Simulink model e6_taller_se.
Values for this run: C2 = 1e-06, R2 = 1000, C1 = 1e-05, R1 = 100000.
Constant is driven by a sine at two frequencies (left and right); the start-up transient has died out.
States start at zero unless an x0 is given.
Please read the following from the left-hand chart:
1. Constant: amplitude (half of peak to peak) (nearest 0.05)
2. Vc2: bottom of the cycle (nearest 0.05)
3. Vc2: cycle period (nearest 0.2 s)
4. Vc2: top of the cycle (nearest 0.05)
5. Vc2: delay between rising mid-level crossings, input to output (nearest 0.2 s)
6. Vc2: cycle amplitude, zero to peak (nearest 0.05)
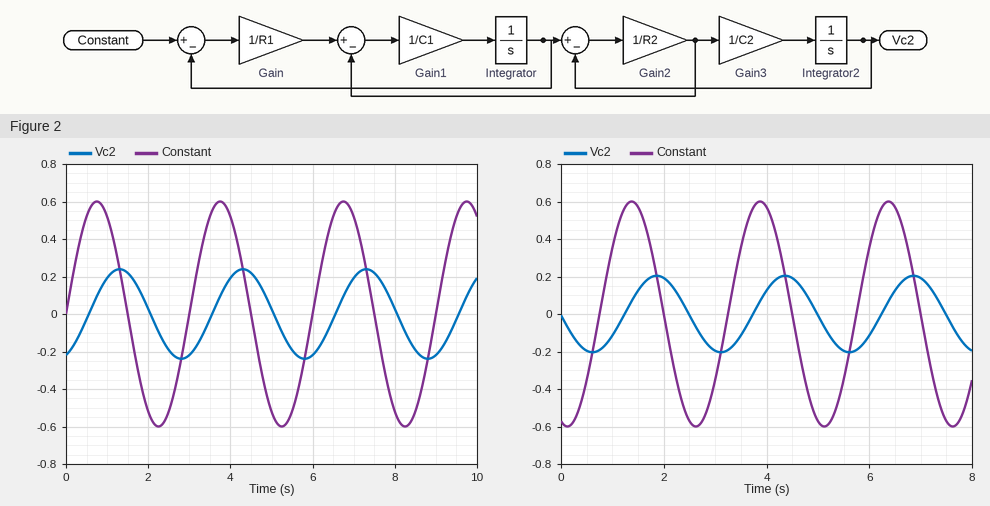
0.60
-0.25
3.0 s
0.25
0.6 s
0.25
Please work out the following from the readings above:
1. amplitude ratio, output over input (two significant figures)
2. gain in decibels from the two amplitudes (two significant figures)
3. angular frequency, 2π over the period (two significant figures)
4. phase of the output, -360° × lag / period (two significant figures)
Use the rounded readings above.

0.42
-7.6 dB
2.1 rad/s
-72°
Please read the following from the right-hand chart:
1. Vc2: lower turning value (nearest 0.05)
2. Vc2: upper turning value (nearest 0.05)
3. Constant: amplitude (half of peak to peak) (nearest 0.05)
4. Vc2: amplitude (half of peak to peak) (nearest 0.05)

-0.20
0.20
0.60
0.20
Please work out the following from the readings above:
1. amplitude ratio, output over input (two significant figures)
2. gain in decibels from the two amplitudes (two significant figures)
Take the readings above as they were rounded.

0.33
-9.5 dB
